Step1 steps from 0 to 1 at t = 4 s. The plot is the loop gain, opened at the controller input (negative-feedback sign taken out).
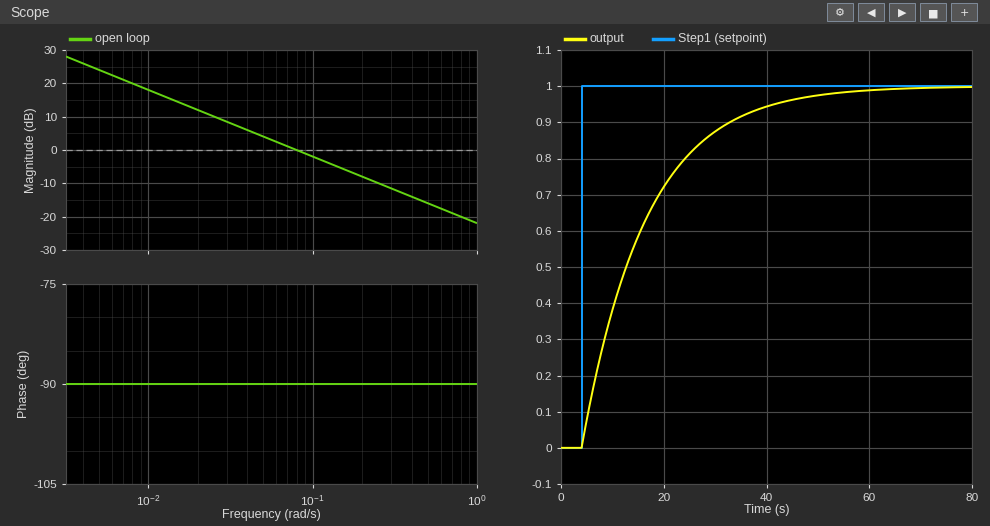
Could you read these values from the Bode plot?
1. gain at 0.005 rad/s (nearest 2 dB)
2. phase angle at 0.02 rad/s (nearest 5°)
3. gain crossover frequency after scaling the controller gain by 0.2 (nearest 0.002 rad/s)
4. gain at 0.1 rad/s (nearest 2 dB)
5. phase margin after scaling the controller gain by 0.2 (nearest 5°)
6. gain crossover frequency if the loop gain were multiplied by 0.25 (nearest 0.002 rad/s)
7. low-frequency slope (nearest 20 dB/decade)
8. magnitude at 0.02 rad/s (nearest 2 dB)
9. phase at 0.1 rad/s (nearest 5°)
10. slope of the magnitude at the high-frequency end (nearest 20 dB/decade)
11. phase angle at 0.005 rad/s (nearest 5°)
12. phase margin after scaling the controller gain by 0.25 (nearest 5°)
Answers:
24 dB
-90°
0.016 rad/s
-2 dB
90°
0.020 rad/s
-20 dB/decade
12 dB
-90°
-20 dB/decade
-90°
90°
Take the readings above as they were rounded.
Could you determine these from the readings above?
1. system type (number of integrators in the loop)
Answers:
1
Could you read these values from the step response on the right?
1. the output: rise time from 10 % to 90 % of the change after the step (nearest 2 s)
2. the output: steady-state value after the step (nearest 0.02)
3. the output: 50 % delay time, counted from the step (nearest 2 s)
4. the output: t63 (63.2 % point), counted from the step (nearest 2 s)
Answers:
28 s
1.00
8 s
12 s
